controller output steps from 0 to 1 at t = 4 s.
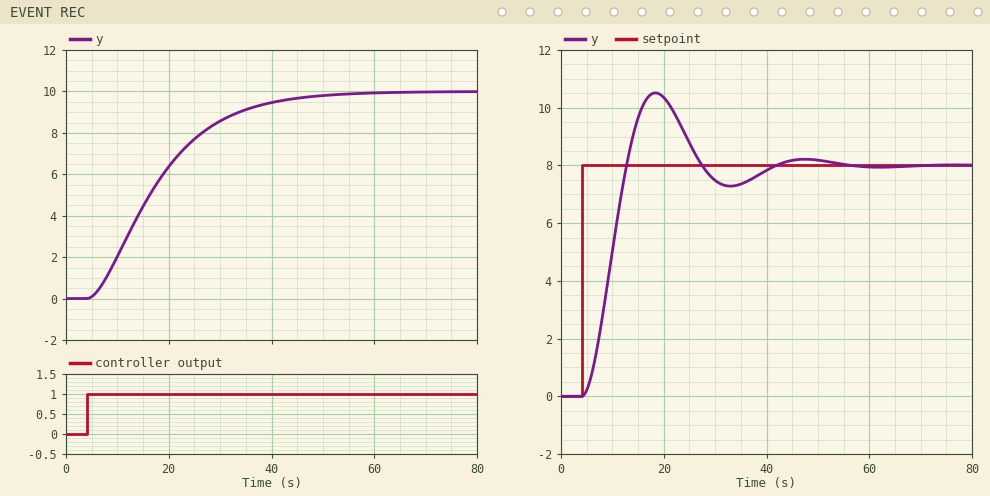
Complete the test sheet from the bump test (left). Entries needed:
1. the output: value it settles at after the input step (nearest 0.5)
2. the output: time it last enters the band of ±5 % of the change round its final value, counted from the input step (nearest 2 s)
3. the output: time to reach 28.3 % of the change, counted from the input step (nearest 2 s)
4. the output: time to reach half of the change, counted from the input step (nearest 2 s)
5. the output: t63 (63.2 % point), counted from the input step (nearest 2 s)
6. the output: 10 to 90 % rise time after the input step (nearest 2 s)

10.0
36 s
8 s
12 s
16 s
26 s
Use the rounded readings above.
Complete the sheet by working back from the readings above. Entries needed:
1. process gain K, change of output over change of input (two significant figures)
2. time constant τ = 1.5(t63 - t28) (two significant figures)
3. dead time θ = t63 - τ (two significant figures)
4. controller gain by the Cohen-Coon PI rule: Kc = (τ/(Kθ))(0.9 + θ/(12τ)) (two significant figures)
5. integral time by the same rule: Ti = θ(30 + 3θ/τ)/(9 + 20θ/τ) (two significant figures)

10
12 s
4.0 s
0.28
7.9 s
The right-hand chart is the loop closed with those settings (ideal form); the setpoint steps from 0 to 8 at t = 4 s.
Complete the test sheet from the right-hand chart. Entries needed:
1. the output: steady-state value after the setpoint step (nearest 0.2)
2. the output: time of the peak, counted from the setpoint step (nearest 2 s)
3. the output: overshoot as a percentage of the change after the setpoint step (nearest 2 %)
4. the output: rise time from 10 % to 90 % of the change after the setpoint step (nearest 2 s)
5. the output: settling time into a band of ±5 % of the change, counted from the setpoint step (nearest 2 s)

8.0
14 s
32 %
6 s
34 s
